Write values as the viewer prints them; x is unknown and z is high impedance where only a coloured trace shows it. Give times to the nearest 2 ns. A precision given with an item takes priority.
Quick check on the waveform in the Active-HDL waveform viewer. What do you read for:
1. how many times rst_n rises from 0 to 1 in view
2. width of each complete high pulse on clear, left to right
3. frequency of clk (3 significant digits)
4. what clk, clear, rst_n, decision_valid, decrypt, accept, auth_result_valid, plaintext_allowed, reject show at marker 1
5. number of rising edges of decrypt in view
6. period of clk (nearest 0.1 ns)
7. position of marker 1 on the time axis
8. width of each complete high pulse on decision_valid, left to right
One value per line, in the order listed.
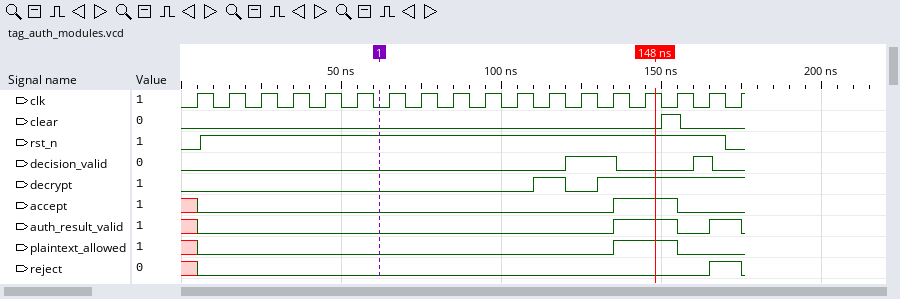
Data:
1
6 ns
100 MHz
clk=0, clear=0, rst_n=1, decision_valid=0, decrypt=0, accept=0, auth_result_valid=0, plaintext_allowed=0, reject=0
2
10 ns
62 ns
16 ns, 6 ns
